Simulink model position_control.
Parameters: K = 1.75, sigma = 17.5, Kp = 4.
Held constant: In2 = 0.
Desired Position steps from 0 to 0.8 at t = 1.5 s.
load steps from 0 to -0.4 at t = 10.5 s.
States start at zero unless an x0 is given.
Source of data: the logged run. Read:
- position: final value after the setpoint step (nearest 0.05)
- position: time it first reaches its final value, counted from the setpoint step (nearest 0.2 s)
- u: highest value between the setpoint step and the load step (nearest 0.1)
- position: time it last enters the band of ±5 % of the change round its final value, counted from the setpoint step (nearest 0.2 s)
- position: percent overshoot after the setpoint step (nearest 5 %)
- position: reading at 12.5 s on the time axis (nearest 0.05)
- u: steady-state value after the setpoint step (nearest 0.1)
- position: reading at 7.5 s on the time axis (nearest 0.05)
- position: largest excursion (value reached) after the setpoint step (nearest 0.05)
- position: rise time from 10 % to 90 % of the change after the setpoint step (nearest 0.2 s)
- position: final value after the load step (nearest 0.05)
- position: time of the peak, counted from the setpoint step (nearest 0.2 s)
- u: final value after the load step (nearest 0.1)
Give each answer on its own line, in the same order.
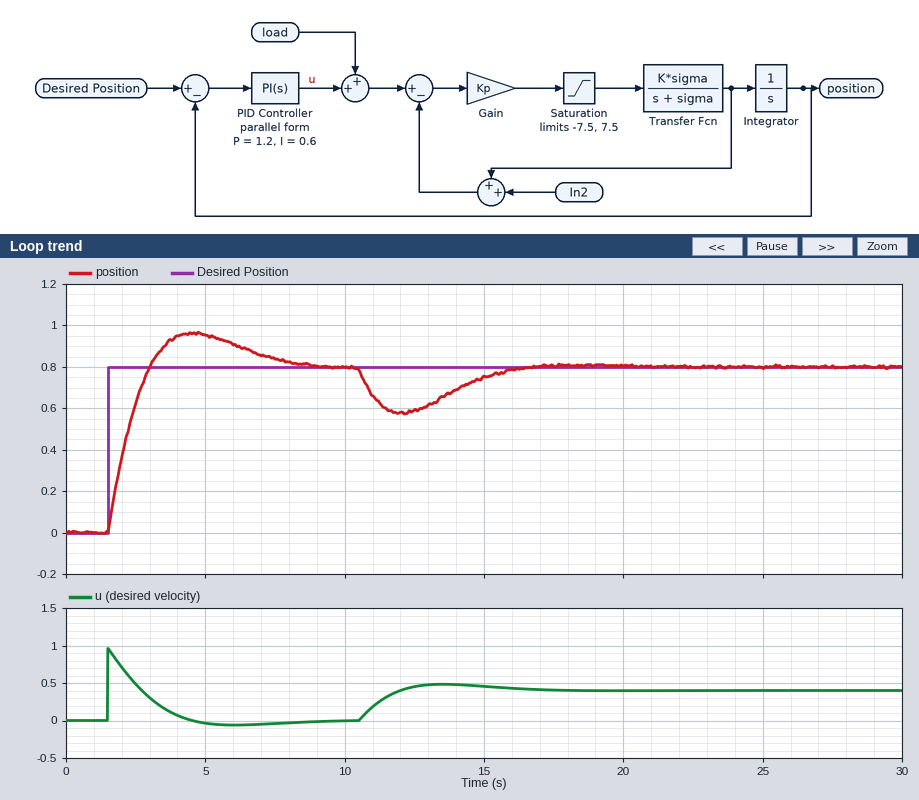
0.80
1.6 s
1.0
6.0 s
20 %
0.60
0.0
0.85
0.95
1.2 s
0.80
3.0 s
0.4
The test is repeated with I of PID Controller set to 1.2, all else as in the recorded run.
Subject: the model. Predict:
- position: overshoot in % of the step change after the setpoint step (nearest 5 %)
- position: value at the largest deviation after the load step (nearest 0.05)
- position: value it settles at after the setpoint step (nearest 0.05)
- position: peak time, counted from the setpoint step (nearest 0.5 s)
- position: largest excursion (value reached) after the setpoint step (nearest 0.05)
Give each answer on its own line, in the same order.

30 %
0.60
0.80
2.5 s
1.05
